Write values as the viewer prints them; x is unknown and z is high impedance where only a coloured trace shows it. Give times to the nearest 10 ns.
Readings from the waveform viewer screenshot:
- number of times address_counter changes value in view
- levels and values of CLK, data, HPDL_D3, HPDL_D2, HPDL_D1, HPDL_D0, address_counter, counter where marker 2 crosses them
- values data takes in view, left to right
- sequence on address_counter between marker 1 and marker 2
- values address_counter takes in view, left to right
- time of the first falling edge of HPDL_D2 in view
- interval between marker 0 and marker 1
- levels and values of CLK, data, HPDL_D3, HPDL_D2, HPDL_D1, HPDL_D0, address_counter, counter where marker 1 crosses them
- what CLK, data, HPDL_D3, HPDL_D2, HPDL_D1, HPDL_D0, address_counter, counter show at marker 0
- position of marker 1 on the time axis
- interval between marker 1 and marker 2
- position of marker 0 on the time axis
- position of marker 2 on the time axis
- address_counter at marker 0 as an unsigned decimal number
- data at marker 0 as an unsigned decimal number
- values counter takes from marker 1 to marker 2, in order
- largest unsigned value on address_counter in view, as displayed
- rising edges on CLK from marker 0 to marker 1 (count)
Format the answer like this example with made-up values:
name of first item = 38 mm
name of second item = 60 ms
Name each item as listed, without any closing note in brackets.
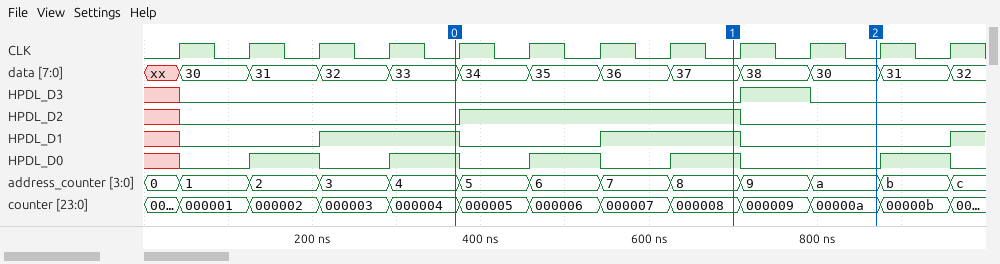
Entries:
number of times address_counter changes value in view = 12
levels and values of CLK, data, HPDL_D3, HPDL_D2, HPDL_D1, HPDL_D0, address_counter, counter where marker 2 crosses them = CLK=0, data=30, HPDL_D3=0, HPDL_D2=0, HPDL_D1=0, HPDL_D0=0, address_counter=a, counter=00000a
values data takes in view, left to right = xx, 30, 31, 32, 33, 34, 35, 36, 37, 38, 30, 31, 32
sequence on address_counter between marker 1 and marker 2 = 8, 9, a
values address_counter takes in view, left to right = 0, 1, 2, 3, 4, 5, 6, 7, 8, 9, a, b, c
time of the first falling edge of HPDL_D2 in view = 710 ns
interval between marker 0 and marker 1 = 330 ns
levels and values of CLK, data, HPDL_D3, HPDL_D2, HPDL_D1, HPDL_D0, address_counter, counter where marker 1 crosses them = CLK=0, data=37, HPDL_D3=0, HPDL_D2=1, HPDL_D1=1, HPDL_D0=1, address_counter=8, counter=000008
what CLK, data, HPDL_D3, HPDL_D2, HPDL_D1, HPDL_D0, address_counter, counter show at marker 0 = CLK=0, data=33, HPDL_D3=0, HPDL_D2=0, HPDL_D1=1, HPDL_D0=1, address_counter=4, counter=000004
position of marker 1 on the time axis = 700 ns
interval between marker 1 and marker 2 = 170 ns
position of marker 0 on the time axis = 370 ns
position of marker 2 on the time axis = 870 ns
address_counter at marker 0 as an unsigned decimal number = 4
data at marker 0 as an unsigned decimal number = 51
values counter takes from marker 1 to marker 2, in order = 000008, 000009, 00000a
largest unsigned value on address_counter in view, as displayed = c
rising edges on CLK from marker 0 to marker 1 = 4
